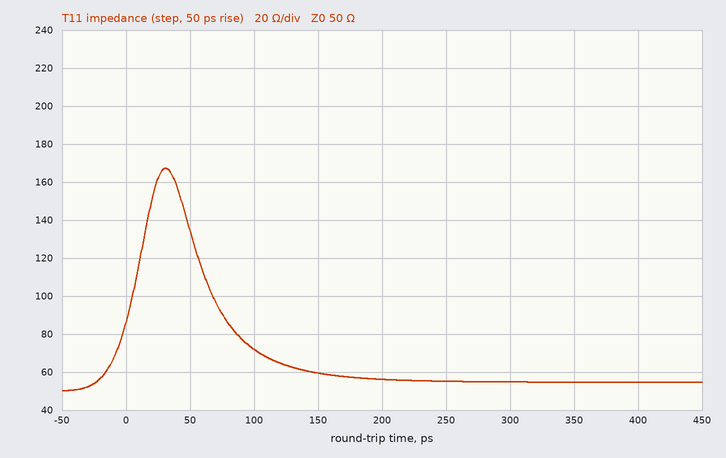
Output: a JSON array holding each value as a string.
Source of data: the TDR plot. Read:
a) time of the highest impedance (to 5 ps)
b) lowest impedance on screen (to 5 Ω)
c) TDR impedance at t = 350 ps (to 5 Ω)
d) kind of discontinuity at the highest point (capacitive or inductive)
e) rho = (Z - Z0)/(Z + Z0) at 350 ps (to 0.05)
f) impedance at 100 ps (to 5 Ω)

["30 ps", "50 Ω", "55 Ω", "inductive", "+0.05", "70 Ω"]
